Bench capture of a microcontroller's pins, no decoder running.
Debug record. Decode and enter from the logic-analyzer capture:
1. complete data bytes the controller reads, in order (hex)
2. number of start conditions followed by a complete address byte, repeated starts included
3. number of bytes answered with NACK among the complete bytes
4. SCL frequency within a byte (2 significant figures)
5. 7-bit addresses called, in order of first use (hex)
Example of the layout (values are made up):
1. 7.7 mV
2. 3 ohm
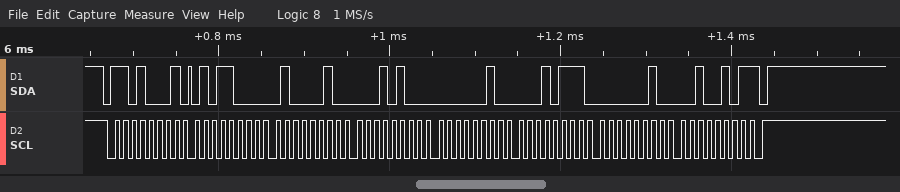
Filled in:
1. 58 42 14 02 17 02 25
2. 1
3. 1
4. 100 kHz
5. 0x68
